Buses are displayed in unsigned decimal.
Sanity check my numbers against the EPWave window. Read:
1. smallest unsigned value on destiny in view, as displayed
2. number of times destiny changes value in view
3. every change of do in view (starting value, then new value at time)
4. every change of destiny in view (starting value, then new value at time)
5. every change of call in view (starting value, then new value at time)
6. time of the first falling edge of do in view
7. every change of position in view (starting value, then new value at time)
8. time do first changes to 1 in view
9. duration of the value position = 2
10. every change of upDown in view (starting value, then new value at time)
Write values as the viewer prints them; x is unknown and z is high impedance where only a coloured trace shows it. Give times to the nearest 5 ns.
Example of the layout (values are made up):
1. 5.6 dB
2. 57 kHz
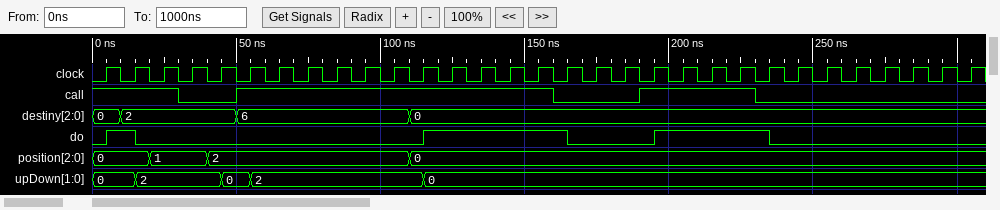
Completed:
1. 0
2. 3
3. 0, 1 at 5 ns, 0 at 15 ns, 1 at 115 ns, 0 at 165 ns, 1 at 195 ns, 0 at 235 ns
4. 0, 2 at 10 ns, 6 at 50 ns, 0 at 110 ns
5. 1, 0 at 30 ns, 1 at 50 ns, 0 at 160 ns, 1 at 190 ns, 0 at 230 ns
6. 15 ns
7. 0, 1 at 20 ns, 2 at 40 ns, 0 at 110 ns
8. 5 ns
9. 70 ns
10. 0, 2 at 15 ns, 0 at 45 ns, 2 at 55 ns, 0 at 115 ns
